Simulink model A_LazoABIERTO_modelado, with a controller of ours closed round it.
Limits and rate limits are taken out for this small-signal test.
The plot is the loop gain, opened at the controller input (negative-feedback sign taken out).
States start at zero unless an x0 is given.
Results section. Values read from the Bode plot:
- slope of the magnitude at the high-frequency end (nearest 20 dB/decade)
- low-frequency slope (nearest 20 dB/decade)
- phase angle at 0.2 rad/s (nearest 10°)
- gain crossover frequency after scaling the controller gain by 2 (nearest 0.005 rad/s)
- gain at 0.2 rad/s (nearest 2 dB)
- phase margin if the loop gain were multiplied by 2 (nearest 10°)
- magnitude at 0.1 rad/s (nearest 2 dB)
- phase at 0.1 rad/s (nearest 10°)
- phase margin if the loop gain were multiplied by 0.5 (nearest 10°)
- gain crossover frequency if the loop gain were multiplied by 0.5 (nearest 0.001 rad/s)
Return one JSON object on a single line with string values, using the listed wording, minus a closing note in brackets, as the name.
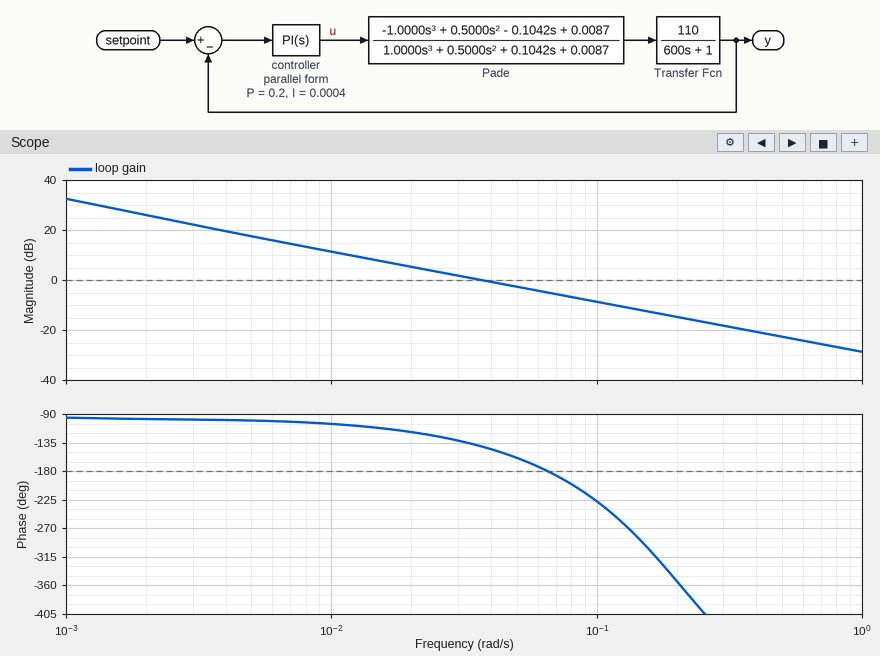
{"slope of the magnitude at the high-frequency end": "-20 dB/decade", "low-frequency slope": "-20 dB/decade", "phase angle at 0.2 rad/s": "-350°", "gain crossover frequency after scaling the controller gain by 2": "0.075 rad/s", "gain at 0.2 rad/s": "-14 dB", "phase margin if the loop gain were multiplied by 2": "-10°", "magnitude at 0.1 rad/s": "-8 dB", "phase at 0.1 rad/s": "-230°", "phase margin if the loop gain were multiplied by 0.5": "60°", "gain crossover frequency if the loop gain were multiplied by 0.5": "0.018 rad/s"}
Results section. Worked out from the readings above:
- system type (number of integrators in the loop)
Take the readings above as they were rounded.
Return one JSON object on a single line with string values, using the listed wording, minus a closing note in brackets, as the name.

{"system type": "1"}
